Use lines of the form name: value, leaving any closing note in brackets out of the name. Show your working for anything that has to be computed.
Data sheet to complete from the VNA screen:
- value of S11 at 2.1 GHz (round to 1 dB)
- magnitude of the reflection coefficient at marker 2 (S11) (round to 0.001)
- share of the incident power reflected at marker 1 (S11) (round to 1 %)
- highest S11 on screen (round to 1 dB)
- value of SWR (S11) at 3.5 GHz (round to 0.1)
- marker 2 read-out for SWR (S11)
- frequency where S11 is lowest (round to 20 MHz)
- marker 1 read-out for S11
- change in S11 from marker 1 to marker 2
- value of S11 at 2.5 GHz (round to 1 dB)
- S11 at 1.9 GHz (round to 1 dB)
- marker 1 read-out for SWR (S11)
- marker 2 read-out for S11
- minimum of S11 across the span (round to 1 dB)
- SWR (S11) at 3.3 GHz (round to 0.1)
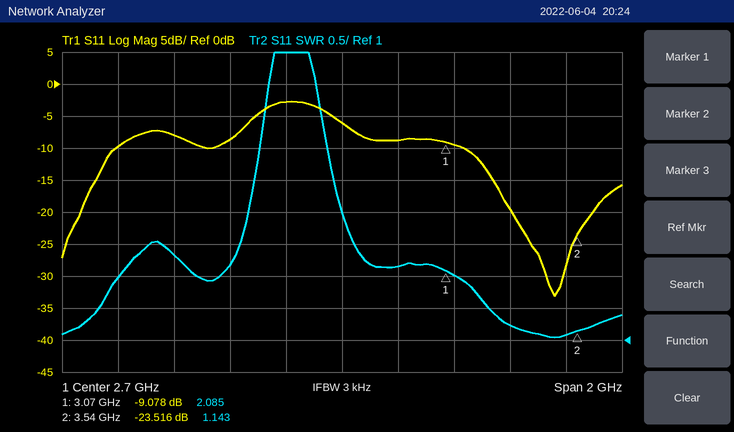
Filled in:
value of S11 at 2.1 GHz: -8 dB
magnitude of the reflection coefficient at marker 2 (S11): 10^(-23.516/20) ≈ 0.067
share of the incident power reflected at marker 1 (S11): 10^(-9.078/10) ≈ 12 %
highest S11 on screen: -3 dB
value of SWR (S11) at 3.5 GHz: 1.1
marker 2 read-out for SWR: 1.143
frequency where S11 is lowest: 3.46 GHz
marker 1 read-out for S11: -9.078 dB
change in S11 from marker 1 to marker 2: -23.516 − (-9.078) = -14.438 dB
value of S11 at 2.5 GHz: -3 dB
S11 at 1.9 GHz: -10 dB
marker 1 read-out for SWR: 2.085
marker 2 read-out for S11: -23.516 dB
minimum of S11 across the span: -33 dB
SWR (S11) at 3.3 GHz: 1.2
